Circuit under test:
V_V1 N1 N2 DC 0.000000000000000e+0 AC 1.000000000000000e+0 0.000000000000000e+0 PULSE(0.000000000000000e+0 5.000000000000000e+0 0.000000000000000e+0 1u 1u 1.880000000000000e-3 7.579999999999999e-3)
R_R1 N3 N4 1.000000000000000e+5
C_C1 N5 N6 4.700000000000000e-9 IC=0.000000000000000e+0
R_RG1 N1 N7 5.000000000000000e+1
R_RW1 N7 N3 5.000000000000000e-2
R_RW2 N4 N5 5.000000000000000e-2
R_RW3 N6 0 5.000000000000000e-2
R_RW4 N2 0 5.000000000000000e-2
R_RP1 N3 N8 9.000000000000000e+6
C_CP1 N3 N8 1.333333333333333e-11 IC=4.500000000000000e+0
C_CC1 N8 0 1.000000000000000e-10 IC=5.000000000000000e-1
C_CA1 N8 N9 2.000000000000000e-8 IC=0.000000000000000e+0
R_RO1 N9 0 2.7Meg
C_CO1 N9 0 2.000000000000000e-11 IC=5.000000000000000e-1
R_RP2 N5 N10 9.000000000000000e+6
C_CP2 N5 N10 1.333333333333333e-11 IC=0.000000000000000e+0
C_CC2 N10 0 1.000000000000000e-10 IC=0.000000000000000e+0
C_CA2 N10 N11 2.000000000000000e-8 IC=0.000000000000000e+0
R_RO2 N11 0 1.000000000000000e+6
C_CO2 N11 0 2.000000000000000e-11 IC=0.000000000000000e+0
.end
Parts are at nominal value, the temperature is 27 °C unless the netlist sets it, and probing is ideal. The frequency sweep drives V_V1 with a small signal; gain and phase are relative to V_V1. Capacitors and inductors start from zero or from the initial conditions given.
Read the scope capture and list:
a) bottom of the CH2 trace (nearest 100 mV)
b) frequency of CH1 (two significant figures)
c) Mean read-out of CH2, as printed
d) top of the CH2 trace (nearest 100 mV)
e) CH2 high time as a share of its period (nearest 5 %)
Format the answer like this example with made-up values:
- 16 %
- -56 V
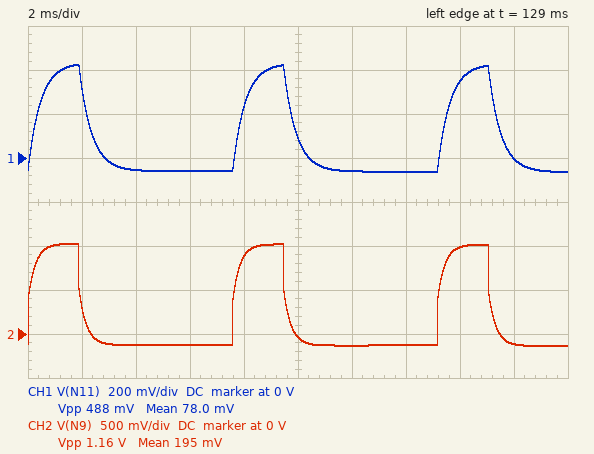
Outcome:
- -100 mV
- 130 Hz
- 195 mV
- 1.0 V
- 25 %
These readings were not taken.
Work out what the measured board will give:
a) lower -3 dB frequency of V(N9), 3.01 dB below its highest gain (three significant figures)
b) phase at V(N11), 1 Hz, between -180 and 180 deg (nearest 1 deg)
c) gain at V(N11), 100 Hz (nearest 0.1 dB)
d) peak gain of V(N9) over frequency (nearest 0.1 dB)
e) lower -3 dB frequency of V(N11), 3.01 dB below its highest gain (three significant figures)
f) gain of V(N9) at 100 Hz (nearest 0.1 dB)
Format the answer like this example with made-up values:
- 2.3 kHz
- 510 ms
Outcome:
- 676 mHz
- 38 deg
- -20.5 dB
- -12.8 dB
- 781 mHz
- -12.9 dB
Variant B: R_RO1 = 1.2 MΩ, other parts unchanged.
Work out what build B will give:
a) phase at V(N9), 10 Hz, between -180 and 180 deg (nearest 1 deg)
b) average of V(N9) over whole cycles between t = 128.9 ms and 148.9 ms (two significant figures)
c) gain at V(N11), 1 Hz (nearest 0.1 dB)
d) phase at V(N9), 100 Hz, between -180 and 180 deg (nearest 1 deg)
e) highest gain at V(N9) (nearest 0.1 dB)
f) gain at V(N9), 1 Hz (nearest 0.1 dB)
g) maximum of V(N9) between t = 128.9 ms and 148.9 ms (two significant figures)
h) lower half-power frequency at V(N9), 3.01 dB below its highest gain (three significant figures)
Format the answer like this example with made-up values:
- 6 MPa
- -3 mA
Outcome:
- 4 deg
- 74 mV
- -22.2 dB
- 0 deg
- -18.6 dB
- -20.7 dB
- 520 mV
- 776 mHz
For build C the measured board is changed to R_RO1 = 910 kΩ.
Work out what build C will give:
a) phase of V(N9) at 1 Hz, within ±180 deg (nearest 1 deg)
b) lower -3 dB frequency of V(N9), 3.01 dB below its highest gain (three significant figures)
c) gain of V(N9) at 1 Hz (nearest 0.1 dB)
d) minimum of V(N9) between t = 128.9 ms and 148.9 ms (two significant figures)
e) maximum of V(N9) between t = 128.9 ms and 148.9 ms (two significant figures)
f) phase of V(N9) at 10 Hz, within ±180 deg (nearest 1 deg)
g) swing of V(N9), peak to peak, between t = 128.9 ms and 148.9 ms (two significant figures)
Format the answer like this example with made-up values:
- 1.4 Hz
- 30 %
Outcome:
- 39 deg
- 973 mHz
- -22.9 dB
- -100 mV
- 450 mV
- 5 deg
- 550 mV
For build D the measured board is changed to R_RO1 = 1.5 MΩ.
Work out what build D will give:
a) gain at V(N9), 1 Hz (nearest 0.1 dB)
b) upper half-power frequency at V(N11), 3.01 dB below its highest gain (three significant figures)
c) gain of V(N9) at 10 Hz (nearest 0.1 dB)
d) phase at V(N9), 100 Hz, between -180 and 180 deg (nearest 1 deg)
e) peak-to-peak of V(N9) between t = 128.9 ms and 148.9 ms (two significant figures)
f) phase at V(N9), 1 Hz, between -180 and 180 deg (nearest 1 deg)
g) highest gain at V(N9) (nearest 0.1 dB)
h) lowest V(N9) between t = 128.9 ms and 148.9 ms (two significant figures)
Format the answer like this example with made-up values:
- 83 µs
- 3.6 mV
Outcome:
- -18.9 dB
- 343 Hz
- -17.0 dB
- -1 deg
- 720 mV
- 37 deg
- -16.9 dB
- -91 mV
